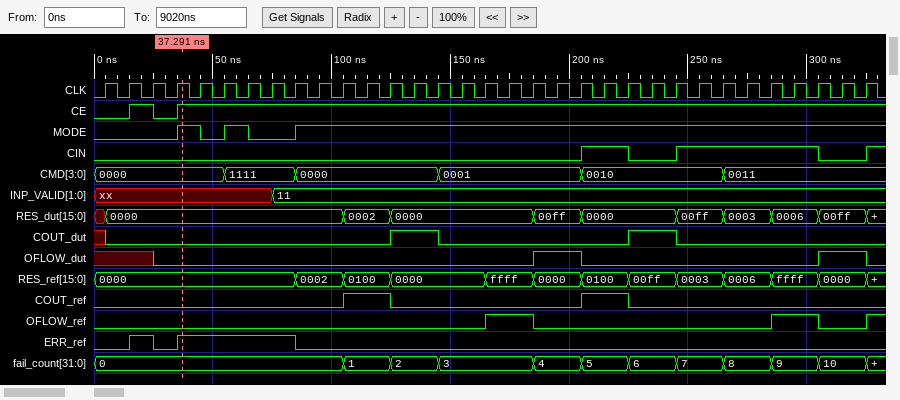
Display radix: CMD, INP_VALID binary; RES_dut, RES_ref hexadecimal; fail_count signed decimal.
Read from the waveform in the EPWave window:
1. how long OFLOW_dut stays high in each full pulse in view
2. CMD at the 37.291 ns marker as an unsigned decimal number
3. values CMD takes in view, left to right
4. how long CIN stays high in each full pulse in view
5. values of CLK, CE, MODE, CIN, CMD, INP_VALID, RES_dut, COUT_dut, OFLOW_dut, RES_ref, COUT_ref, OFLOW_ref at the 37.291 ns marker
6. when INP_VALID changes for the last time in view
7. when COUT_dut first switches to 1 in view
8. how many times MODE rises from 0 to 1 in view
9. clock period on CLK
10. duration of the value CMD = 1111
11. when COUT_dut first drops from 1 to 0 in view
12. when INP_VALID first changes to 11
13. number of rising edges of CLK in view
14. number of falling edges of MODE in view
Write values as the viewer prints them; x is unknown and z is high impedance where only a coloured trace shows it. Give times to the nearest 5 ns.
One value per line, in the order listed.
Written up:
20 ns, 20 ns
0
0000, 1111, 0000, 0001, 0010, 0011
20 ns, 60 ns
CLK=1, CE=1, MODE=1, CIN=0, CMD=0000, INP_VALID=xx, RES_dut=0000, COUT_dut=0, OFLOW_dut=0, RES_ref=0000, COUT_ref=0, OFLOW_ref=0
75 ns
125 ns
3
10 ns
30 ns
145 ns
75 ns
33
2
